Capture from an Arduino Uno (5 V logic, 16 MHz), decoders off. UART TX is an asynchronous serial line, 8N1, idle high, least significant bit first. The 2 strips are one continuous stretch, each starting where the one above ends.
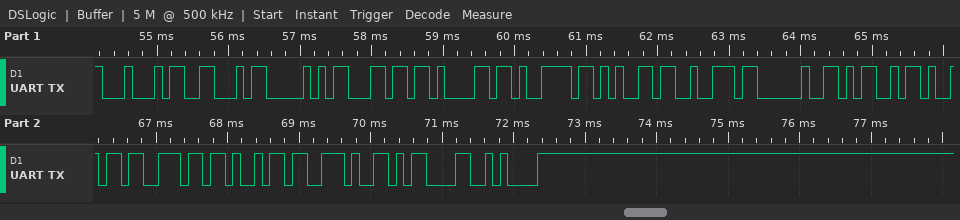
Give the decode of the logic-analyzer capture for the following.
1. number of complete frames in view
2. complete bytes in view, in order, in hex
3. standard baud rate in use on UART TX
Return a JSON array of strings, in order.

["16", "0x44 0x46 0x50 0x6C 0x61 0x79 0x65 0x72 0x20 0x4D 0x69 0x6E 0x69 0x2E 0x0D 0x0A", "9600 baud"]
